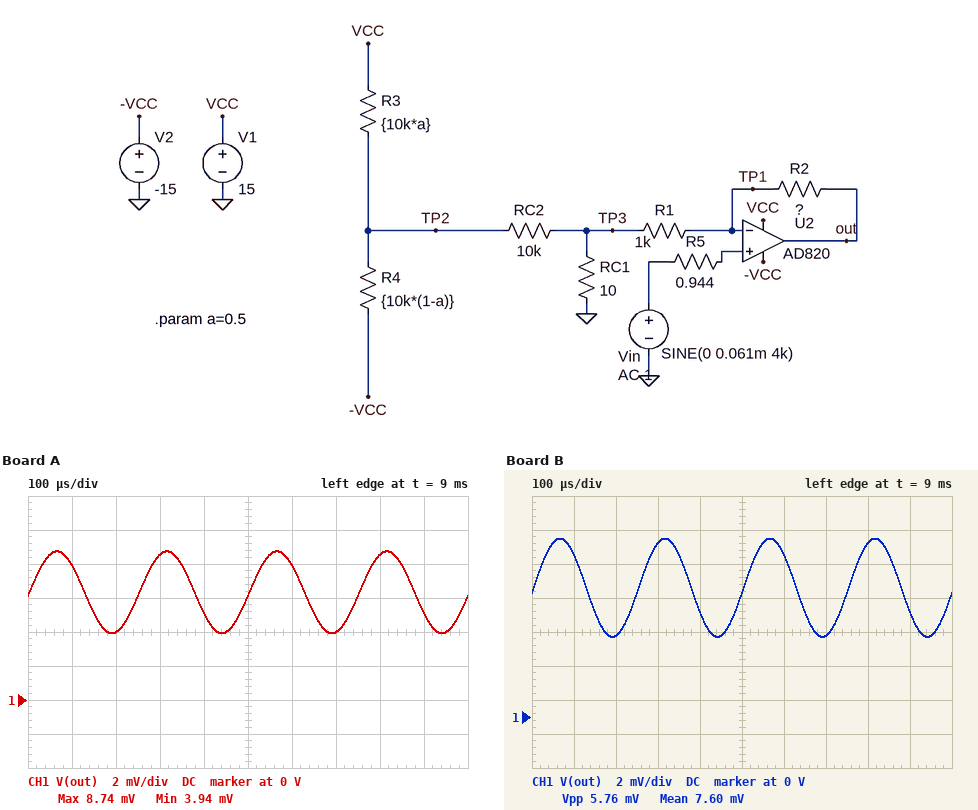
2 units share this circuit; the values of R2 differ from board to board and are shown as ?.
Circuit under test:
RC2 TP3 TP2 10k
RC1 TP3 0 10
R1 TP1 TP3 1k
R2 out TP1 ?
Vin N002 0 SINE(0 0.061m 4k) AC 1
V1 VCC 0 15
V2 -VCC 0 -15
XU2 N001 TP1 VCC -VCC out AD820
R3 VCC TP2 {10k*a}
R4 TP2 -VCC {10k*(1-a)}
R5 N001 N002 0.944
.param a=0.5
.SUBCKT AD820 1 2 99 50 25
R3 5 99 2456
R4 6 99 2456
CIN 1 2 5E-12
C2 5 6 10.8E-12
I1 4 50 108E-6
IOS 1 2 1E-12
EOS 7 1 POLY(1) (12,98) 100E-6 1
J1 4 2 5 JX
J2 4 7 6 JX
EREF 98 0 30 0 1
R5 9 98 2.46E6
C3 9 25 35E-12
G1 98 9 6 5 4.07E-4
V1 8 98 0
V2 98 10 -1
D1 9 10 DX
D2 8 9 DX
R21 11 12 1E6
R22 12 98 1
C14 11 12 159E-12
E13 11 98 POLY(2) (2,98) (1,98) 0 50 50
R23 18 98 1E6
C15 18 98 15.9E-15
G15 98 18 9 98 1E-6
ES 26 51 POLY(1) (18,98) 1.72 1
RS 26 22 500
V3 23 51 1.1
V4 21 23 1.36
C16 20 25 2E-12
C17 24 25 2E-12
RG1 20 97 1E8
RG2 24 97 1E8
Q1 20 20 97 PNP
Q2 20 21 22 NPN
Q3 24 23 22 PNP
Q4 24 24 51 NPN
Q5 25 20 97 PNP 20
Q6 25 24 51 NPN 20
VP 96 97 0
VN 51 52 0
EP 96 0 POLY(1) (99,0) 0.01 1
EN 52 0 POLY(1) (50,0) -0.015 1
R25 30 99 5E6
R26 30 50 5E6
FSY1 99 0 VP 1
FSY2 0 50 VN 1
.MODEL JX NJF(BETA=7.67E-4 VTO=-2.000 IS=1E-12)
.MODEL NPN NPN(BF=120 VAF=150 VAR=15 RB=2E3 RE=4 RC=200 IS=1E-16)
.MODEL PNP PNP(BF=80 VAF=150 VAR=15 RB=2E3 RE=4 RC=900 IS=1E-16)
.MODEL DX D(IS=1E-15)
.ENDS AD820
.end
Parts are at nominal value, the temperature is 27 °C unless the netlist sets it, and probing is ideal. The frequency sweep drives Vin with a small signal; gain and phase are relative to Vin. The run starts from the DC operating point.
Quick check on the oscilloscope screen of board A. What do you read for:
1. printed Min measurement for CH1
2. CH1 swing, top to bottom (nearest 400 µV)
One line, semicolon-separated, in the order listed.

3.94 mV; 4.8 mV
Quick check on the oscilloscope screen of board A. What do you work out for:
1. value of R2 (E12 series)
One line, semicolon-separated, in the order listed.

39 kΩ
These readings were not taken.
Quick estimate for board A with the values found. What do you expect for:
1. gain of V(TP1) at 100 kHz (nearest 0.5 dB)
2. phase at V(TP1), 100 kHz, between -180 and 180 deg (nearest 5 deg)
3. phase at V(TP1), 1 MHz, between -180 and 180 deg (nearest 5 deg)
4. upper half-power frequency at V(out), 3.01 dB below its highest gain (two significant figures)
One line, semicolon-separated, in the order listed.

-7.5 dB; -65 deg; -140 deg; 48 kHz
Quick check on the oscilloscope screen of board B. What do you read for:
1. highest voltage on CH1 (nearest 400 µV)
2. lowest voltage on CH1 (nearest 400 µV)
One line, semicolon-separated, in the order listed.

10.4 mV; 4.8 mV
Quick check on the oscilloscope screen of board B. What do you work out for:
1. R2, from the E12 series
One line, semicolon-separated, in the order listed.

47 kΩ
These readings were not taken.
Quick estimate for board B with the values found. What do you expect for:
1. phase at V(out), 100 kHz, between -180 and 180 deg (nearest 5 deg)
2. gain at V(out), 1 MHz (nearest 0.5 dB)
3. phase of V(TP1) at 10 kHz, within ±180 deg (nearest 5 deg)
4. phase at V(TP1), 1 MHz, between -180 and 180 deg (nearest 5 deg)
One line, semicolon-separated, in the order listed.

-70 deg; 5.0 dB; -15 deg; -160 deg
